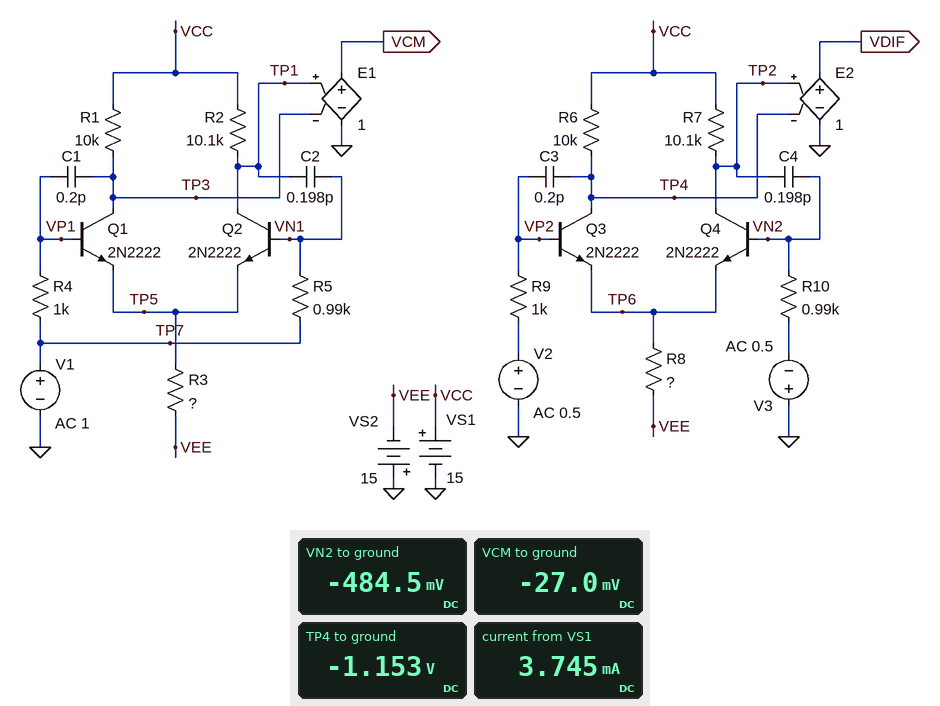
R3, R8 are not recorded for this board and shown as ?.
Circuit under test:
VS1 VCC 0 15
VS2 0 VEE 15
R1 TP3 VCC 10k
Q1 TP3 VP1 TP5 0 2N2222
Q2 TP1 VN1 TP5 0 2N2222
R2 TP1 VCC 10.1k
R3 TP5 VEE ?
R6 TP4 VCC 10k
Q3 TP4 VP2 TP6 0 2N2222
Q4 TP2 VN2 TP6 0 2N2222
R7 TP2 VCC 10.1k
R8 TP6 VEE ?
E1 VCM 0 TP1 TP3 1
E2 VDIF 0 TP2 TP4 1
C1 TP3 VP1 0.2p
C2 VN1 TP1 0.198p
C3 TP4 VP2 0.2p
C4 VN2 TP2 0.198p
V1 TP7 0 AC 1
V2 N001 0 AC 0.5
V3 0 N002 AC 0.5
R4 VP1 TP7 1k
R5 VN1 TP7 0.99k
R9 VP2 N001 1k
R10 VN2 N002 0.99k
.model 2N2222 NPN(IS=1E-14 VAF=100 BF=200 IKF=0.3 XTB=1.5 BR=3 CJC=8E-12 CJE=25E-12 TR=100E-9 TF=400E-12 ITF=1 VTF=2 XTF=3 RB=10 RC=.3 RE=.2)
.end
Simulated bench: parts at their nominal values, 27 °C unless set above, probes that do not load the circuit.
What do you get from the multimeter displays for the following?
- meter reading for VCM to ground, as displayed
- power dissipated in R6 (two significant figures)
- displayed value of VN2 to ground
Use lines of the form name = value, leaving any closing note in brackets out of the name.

meter reading for VCM to ground, as displayed = -27.0 mV
power dissipated in R6 = 26 mW
displayed value of VN2 to ground = -484.5 mV
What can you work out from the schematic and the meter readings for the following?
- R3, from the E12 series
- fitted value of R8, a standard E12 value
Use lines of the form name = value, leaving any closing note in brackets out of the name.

R3, from the E12 series = 27 kΩ
fitted value of R8, a standard E12 value = 3.3 kΩ
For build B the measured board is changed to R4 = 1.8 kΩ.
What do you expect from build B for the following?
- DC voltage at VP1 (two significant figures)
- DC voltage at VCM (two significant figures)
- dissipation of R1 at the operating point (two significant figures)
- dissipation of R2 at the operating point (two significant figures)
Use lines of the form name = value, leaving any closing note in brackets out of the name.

DC voltage at VP1 = -2.1 mV
DC voltage at VCM = -120 mV
dissipation of R1 at the operating point = 680 µW
dissipation of R2 at the operating point = 730 µW
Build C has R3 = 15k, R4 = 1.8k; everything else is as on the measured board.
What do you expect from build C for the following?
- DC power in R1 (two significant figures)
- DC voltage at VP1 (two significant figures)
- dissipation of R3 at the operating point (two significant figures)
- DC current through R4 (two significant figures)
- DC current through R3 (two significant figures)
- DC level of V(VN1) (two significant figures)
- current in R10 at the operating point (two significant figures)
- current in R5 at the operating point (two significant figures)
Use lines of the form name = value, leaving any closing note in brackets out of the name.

DC power in R1 = 2.1 mW
DC voltage at VP1 = -3.8 mV
dissipation of R3 at the operating point = 14 mW
DC current through R4 = 2.1 µA
DC current through R3 = 960 µA
DC level of V(VN1) = -2.2 mV
current in R10 at the operating point = 490 µA
current in R5 at the operating point = 2.2 µA
